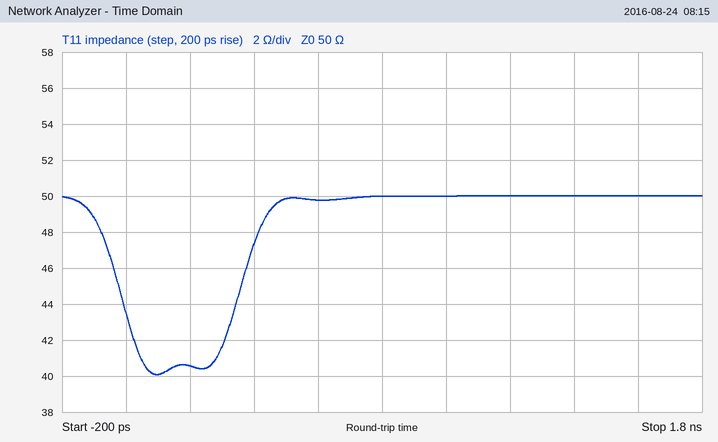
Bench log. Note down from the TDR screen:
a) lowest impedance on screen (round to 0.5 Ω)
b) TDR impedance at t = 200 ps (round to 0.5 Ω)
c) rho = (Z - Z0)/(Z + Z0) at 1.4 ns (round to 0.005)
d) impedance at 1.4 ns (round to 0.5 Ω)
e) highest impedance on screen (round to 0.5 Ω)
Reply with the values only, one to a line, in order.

40.0 Ω
40.5 Ω
0.000
50.0 Ω
50.0 Ω
